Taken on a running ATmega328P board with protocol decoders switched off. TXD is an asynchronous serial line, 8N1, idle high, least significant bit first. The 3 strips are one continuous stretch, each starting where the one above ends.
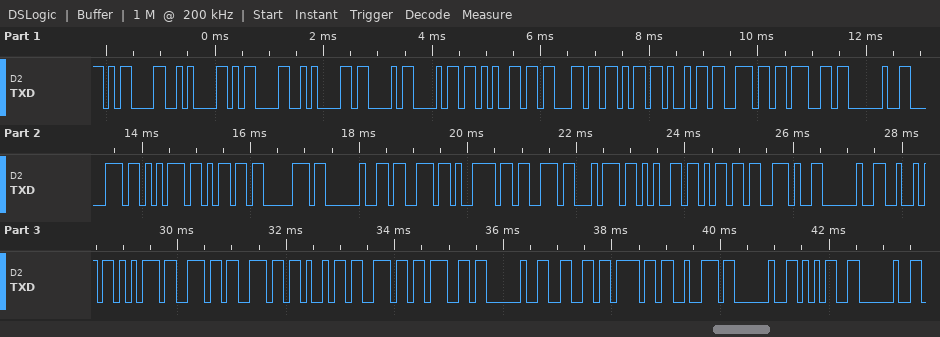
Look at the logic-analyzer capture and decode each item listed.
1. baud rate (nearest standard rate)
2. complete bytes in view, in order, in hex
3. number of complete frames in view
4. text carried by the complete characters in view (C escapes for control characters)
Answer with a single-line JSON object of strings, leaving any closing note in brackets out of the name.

{"baud rate": "9600 baud", "complete bytes in view, in order, in hex": "0x0D 0x0A 0x0D 0x0A 0x43 0x68 0x65 0x63 0x6B 0x69 0x6E 0x67 0x20 0x70 0x75 0x6D 0x70 0x20 0x73 0x79 0x73 0x74 0x65 0x6D 0x2E 0x20 0x52 0x75 0x6E 0x6E 0x69 0x6E 0x67 0x20 0x66 0x6F 0x72 0x20 0x35 0x20", "number of complete frames in view": "40", "text carried by the complete characters in view": "\"\\r\\n\\r\\nChecking pump system. Running for 5 \""}
